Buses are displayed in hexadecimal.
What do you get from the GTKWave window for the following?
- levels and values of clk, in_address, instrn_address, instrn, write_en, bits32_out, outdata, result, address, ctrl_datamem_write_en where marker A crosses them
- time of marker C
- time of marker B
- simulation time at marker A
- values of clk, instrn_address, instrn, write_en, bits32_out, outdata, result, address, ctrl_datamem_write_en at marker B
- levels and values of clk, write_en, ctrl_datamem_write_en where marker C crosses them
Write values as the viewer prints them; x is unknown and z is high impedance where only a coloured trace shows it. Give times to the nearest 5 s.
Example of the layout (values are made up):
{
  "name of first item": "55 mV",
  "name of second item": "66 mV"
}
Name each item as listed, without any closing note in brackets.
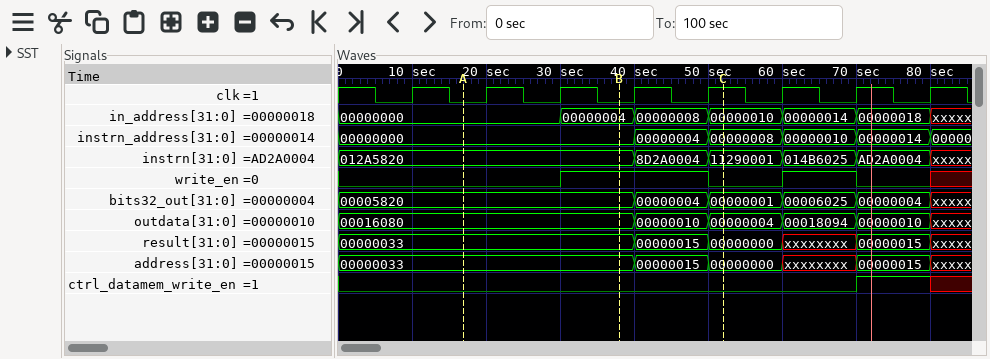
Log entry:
{
  "levels and values of clk, in_address, instrn_address, instrn, write_en, bits32_out, outdata, result, address, ctrl_datamem_write_en where marker A crosses them": "clk=0, in_address=00000000, instrn_address=00000000, instrn=012A5820, write_en=0, bits32_out=00005820, outdata=00016080, result=00000033, address=00000033, ctrl_datamem_write_en=0",
  "time of marker C": "50 s",
  "time of marker B": "40 s",
  "simulation time at marker A": "15 s",
  "values of clk, instrn_address, instrn, write_en, bits32_out, outdata, result, address, ctrl_datamem_write_en at marker B": "clk=0, instrn_address=00000000, instrn=012A5820, write_en=1, bits32_out=00005820, outdata=00016080, result=00000033, address=00000033, ctrl_datamem_write_en=0",
  "levels and values of clk, write_en, ctrl_datamem_write_en where marker C crosses them": "clk=1, write_en=0, ctrl_datamem_write_en=0"
}
